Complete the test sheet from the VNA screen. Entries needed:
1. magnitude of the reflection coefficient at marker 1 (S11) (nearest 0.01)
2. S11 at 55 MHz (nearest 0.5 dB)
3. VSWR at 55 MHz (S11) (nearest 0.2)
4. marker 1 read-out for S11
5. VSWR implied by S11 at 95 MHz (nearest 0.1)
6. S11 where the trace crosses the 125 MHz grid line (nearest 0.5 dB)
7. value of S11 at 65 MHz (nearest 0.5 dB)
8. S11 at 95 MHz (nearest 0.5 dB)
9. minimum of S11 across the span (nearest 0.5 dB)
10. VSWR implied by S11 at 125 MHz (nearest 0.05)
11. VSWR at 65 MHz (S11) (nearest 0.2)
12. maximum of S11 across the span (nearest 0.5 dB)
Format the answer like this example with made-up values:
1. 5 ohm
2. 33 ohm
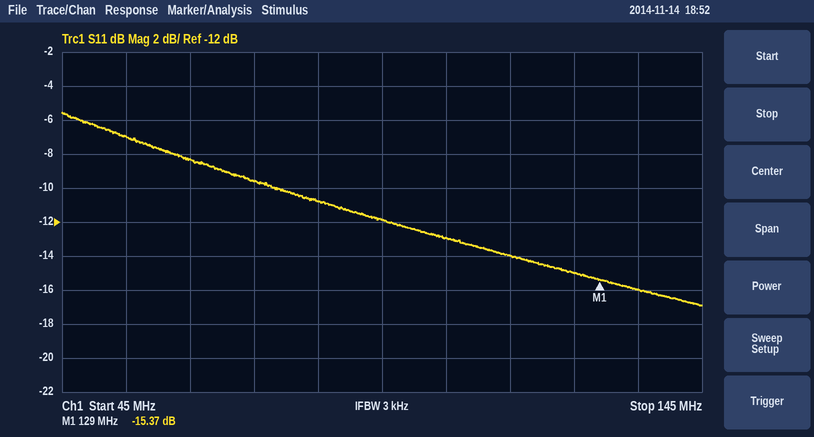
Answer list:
1. 0.17
2. -7.0 dB
3. 2.6
4. -15.37 dB
5. 1.7
6. -15.0 dB
7. -8.5 dB
8. -12.0 dB
9. -17.0 dB
10. 1.45
11. 2.2
12. -5.5 dB
